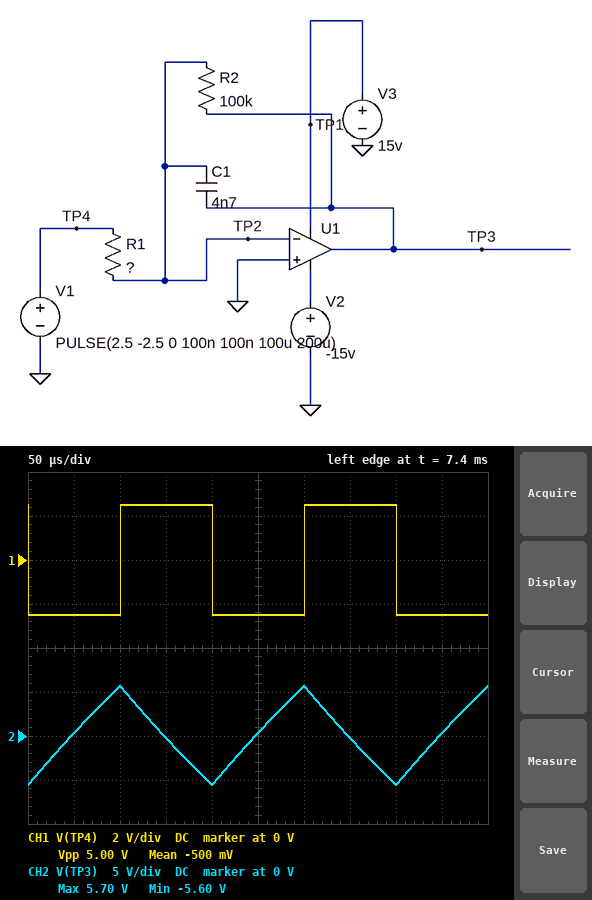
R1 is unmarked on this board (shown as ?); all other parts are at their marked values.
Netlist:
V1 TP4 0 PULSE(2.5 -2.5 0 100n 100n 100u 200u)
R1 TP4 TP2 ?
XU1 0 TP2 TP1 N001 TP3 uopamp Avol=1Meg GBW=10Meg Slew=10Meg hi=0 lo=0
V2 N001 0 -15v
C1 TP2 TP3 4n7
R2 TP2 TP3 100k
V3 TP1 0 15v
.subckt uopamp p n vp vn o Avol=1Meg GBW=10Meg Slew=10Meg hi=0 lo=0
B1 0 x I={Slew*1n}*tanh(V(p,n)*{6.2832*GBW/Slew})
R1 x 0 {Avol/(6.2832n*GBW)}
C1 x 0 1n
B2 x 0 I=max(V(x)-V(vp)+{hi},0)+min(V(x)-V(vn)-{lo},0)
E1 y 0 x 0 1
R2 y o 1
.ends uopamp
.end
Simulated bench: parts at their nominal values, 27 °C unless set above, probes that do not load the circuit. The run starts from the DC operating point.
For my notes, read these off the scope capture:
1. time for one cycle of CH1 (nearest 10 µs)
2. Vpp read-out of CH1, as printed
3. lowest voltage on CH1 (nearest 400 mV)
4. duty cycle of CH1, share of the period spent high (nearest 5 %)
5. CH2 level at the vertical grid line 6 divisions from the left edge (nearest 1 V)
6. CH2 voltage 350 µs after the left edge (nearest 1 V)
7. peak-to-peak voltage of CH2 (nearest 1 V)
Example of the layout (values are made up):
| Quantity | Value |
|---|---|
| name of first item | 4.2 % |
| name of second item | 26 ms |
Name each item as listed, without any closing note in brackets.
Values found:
| Quantity | Value |
|---|---|
| time for one cycle of CH1 | 200 µs |
| Vpp read-out of CH1, as printed | 5.00 V |
| lowest voltage on CH1 | -2.4 V |
| duty cycle of CH1, share of the period spent high | 50 % |
| CH2 level at the vertical grid line 6 divisions from the left edge | 6 V |
| CH2 voltage 350 µs after the left edge | 0 V |
| peak-to-peak voltage of CH2 | 11 V |
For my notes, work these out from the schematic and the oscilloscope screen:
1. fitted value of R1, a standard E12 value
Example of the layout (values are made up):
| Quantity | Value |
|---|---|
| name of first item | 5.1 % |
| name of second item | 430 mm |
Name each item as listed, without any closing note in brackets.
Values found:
| Quantity | Value |
|---|---|
| fitted value of R1, a standard E12 value | 4.7 kΩ |
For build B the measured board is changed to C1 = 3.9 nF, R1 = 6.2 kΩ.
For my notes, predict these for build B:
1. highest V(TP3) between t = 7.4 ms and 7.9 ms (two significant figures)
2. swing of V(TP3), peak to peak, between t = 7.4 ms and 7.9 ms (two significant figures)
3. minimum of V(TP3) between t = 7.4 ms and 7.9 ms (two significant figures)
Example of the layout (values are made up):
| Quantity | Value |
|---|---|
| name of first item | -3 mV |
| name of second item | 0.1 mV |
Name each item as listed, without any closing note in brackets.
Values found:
| Quantity | Value |
|---|---|
| highest V(TP3) between t = 7.4 ms and 7.9 ms | 5.2 V |
| swing of V(TP3), peak to peak, between t = 7.4 ms and 7.9 ms | 10 V |
| minimum of V(TP3) between t = 7.4 ms and 7.9 ms | -5.1 V |
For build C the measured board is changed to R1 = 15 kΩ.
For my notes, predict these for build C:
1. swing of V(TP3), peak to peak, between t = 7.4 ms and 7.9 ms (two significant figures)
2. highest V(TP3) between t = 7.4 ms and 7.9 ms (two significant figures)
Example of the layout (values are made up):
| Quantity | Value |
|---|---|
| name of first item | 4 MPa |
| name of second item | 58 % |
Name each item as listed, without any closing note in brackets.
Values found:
| Quantity | Value |
|---|---|
| swing of V(TP3), peak to peak, between t = 7.4 ms and 7.9 ms | 3.5 V |
| highest V(TP3) between t = 7.4 ms and 7.9 ms | 1.8 V |
